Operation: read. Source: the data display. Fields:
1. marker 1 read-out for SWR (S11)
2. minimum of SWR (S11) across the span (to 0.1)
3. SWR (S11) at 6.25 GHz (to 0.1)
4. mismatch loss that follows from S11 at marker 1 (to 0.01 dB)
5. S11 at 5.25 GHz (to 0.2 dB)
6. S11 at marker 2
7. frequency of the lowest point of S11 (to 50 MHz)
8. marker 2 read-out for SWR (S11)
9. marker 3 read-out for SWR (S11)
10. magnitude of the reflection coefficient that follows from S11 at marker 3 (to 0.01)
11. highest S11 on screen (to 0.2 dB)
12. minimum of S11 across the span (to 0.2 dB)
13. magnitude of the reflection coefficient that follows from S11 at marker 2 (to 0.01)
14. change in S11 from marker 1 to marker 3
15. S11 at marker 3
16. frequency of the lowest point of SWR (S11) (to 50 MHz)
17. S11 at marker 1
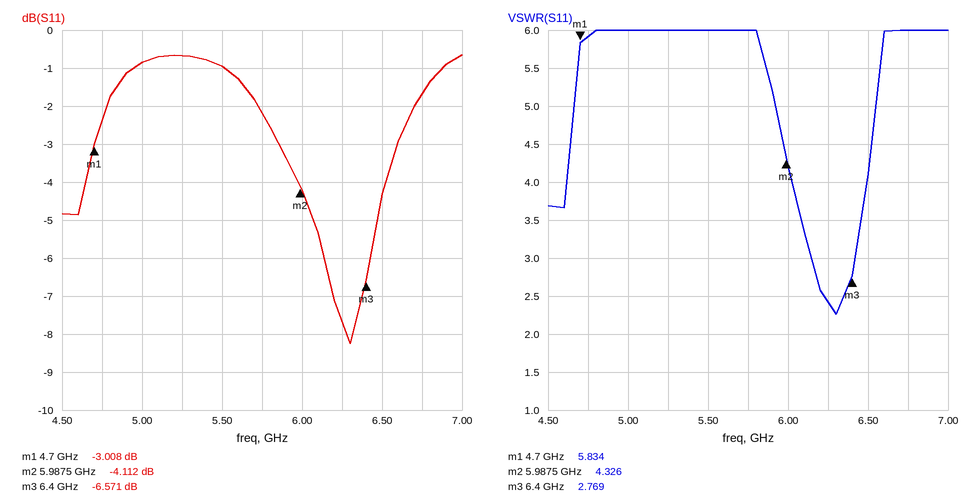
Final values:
5.834
2.3
2.4
3.01 dB
-0.6 dB
-4.112 dB
6.30 GHz
4.326
2.769
0.47
-0.6 dB
-8.2 dB
0.62
-3.563 dB
-6.571 dB
6.30 GHz
-3.008 dB
